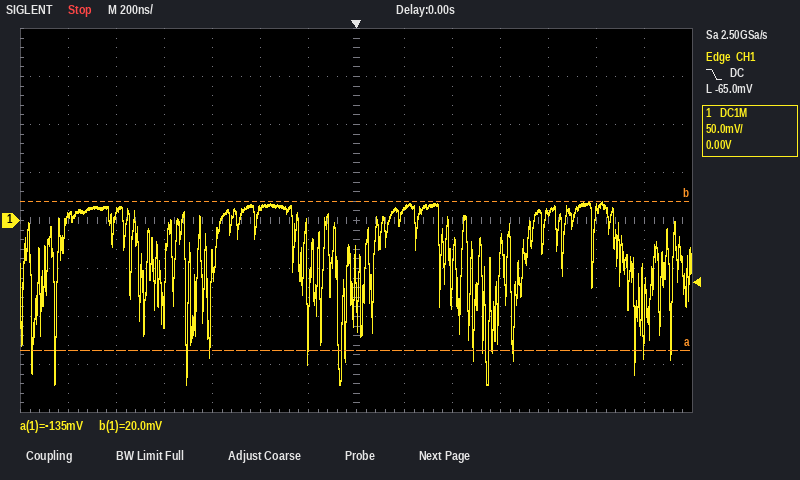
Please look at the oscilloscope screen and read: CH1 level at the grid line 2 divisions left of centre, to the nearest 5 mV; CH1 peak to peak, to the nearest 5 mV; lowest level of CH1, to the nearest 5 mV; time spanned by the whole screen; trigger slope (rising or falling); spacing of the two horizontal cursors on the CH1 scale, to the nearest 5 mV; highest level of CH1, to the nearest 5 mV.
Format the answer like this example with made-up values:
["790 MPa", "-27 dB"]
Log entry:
["10 mV", "190 mV", "-170 mV", "2.8 µs", "falling", "155 mV", "20 mV"]
